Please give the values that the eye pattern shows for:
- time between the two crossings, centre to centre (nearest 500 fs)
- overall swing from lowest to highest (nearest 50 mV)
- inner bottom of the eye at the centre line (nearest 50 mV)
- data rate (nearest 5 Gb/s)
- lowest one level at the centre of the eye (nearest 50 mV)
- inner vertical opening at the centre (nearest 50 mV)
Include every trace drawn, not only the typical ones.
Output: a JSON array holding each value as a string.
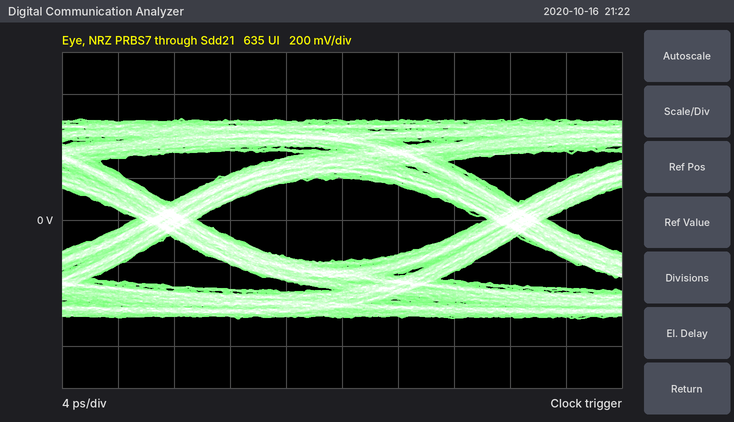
["25.0 ps", "950 mV", "-200 mV", "40 Gb/s", "200 mV", "400 mV"]
